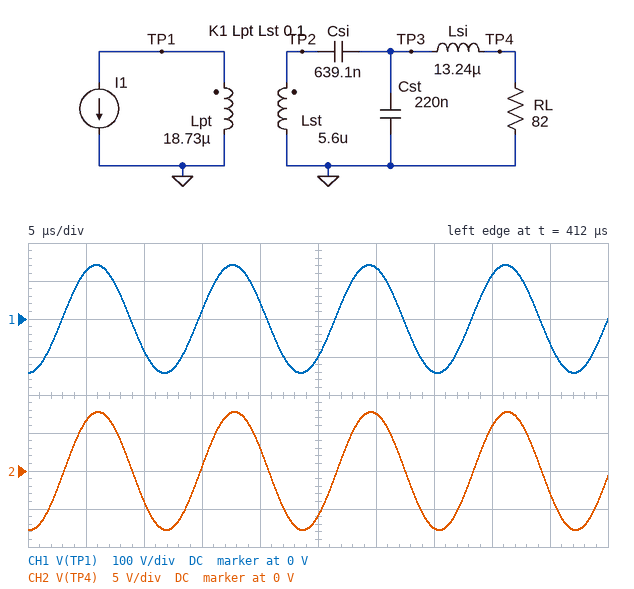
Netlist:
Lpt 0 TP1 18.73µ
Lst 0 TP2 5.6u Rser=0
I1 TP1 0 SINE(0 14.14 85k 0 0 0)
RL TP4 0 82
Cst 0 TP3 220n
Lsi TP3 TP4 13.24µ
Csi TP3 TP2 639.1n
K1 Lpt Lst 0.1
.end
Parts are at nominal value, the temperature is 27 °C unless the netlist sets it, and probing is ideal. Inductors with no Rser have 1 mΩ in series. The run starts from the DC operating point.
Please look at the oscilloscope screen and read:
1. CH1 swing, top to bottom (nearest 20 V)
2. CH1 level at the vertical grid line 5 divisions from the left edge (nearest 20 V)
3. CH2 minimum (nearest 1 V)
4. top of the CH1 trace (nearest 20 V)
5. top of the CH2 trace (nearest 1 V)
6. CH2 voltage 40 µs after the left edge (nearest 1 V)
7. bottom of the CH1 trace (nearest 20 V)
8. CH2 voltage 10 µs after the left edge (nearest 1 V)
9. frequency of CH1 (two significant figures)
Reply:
280 V
-100 V
-8 V
140 V
8 V
6 V
-140 V
-4 V
85 kHz
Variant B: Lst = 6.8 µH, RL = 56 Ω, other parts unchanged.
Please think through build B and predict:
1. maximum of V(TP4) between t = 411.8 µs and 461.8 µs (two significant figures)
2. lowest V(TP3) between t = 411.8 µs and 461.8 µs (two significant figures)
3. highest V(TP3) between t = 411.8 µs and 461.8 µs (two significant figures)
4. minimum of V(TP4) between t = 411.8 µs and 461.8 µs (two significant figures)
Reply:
9.2 V
-9.3 V
9.3 V
-9.2 V
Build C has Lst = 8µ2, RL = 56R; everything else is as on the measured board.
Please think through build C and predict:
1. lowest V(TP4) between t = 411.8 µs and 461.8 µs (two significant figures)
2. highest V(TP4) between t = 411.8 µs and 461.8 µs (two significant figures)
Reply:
-11 V
11 V
